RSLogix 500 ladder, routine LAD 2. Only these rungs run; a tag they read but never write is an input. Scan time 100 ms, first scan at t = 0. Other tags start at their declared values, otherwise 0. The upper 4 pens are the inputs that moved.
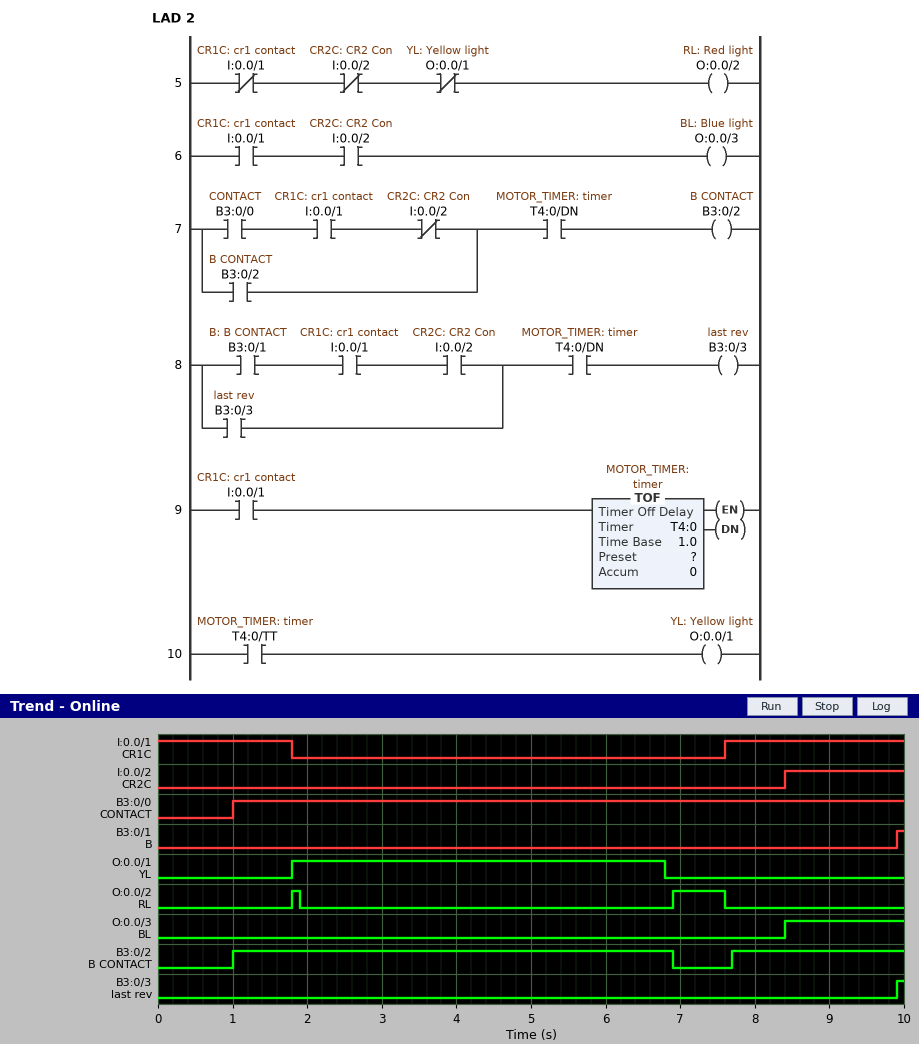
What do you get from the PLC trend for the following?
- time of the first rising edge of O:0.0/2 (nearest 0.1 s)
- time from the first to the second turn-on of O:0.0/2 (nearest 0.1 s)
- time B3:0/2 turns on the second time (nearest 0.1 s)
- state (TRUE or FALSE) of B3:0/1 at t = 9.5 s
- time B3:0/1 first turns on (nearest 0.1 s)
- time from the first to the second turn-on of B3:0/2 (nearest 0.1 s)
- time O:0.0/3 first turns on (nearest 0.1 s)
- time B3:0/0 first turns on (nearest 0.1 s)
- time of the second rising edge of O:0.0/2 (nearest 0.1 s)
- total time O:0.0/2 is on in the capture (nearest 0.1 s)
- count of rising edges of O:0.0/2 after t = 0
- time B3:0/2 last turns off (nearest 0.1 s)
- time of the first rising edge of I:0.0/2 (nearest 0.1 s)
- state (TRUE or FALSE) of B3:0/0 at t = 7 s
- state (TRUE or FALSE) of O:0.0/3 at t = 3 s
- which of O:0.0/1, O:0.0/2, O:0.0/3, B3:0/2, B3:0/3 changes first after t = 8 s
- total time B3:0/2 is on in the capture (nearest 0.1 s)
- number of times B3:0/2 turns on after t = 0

1.8 s
5.1 s
7.7 s
FALSE
9.9 s
6.7 s
8.4 s
1.0 s
6.9 s
0.8 s
2
6.9 s
8.4 s
TRUE
FALSE
O:0.0/3
8.2 s
2
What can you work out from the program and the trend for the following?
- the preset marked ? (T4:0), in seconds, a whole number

5 s
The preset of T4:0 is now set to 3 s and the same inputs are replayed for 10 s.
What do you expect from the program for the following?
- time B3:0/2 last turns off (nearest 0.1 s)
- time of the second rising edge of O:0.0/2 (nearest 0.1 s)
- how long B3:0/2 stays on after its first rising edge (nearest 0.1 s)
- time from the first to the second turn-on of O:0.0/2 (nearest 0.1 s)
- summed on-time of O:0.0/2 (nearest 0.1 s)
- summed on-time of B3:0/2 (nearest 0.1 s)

4.9 s
4.9 s
3.9 s
3.1 s
2.8 s
6.2 s
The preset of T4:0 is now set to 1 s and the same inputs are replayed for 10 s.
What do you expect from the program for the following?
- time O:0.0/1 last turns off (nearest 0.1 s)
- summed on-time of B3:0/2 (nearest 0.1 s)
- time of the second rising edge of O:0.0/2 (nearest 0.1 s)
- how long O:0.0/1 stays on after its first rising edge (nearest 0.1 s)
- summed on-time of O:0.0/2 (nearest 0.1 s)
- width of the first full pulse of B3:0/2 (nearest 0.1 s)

2.8 s
4.2 s
2.9 s
1.0 s
4.8 s
1.9 s
